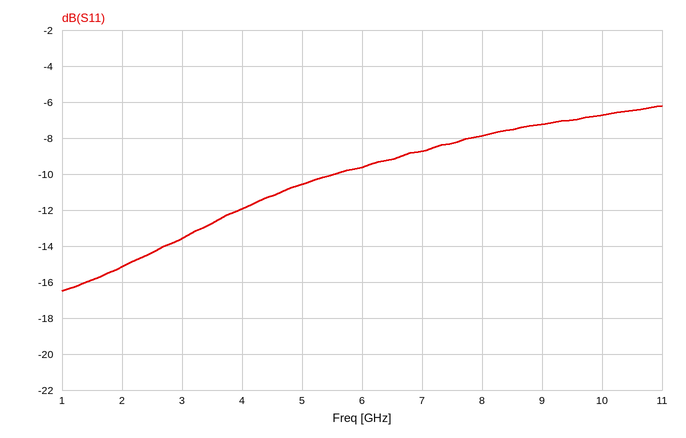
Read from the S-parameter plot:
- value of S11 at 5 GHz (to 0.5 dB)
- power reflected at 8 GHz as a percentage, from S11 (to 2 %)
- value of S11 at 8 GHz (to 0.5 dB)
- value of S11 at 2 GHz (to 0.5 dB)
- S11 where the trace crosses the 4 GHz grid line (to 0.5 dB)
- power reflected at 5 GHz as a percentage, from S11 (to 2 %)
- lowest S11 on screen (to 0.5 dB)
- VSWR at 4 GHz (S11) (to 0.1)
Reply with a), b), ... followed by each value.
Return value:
a) -10.5 dB
b) 16 %
c) -8.0 dB
d) -15.0 dB
e) -12.0 dB
f) 8 %
g) -16.5 dB
h) 1.7
